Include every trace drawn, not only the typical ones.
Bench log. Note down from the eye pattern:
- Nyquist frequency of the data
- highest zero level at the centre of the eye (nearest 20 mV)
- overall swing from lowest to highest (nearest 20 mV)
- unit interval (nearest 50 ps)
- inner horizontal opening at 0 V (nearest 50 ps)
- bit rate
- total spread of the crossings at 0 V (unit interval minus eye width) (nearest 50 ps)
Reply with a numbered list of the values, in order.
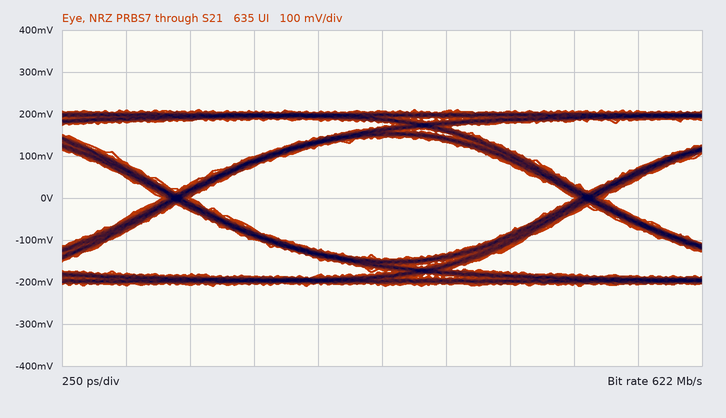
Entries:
1. 311 MHz
2. -140 mV
3. 420 mV
4. 1.60 ns
5. 1.50 ns
6. 622 Mb/s
7. 100 ps
